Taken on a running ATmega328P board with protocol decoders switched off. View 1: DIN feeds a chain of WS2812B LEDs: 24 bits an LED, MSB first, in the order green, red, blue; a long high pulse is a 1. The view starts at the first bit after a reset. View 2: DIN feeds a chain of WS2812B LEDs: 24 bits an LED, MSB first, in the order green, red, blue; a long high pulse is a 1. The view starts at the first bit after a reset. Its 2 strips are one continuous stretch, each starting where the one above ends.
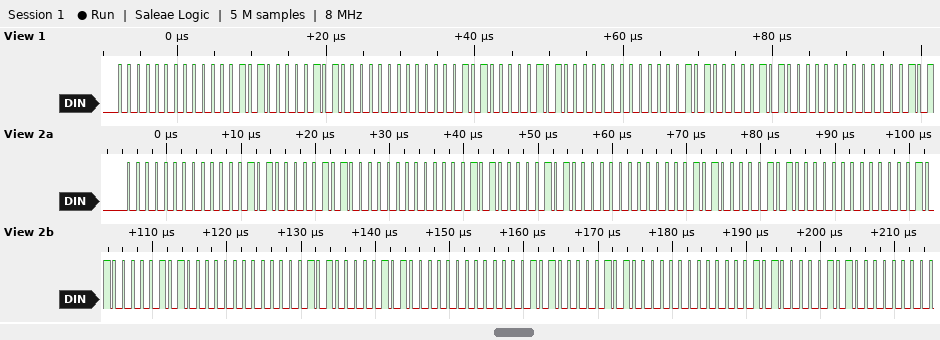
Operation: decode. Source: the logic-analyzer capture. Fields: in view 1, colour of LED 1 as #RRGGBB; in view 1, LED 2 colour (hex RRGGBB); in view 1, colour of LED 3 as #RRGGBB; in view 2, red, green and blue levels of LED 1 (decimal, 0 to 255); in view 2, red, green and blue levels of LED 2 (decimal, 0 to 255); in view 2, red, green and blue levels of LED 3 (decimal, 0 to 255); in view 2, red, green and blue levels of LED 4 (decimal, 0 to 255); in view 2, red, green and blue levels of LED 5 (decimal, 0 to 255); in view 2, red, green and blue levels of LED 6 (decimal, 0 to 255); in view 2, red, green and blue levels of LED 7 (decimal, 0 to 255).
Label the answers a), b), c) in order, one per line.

a) #050005
b) #050005
c) #050005
d) 5, 0, 5
e) 5, 0, 5
f) 5, 0, 5
g) 5, 0, 5
h) 5, 0, 5
i) 5, 0, 5
j) 5, 0, 5
